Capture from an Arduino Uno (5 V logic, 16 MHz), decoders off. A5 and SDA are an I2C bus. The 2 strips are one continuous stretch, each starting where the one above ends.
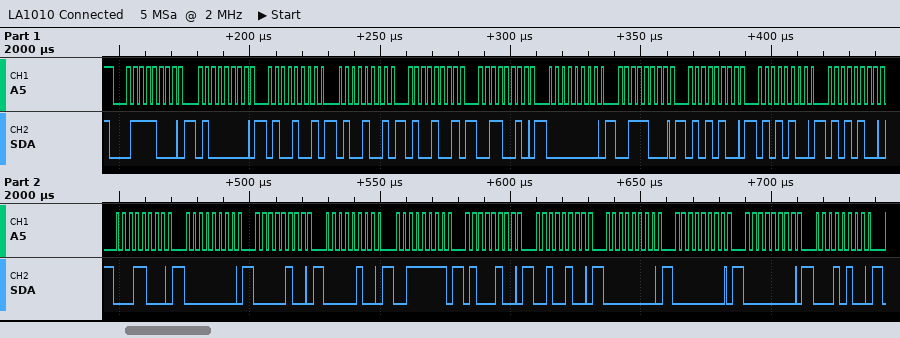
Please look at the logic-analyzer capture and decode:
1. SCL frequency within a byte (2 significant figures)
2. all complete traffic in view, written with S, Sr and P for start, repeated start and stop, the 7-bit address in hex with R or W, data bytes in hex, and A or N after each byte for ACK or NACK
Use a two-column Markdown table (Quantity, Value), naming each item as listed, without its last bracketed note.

| Quantity | Value |
|---|---|
| SCL frequency within a byte | 400 kHz |
| all complete traffic in view, written with S, Sr and P for start, repeated start and stop, the 7-bit address in hex with R or W, data bytes in hex, and A or N after each byte for ACK or NACK | S 3CW A 40 A 49 A 49 A 49 A 32 A 00 A 38 A 54 A 54 A 54 A 18 A 00 A 04 A 04 A 3F A 44 A 24 A 00 A 00 A 00 A 14 A |
